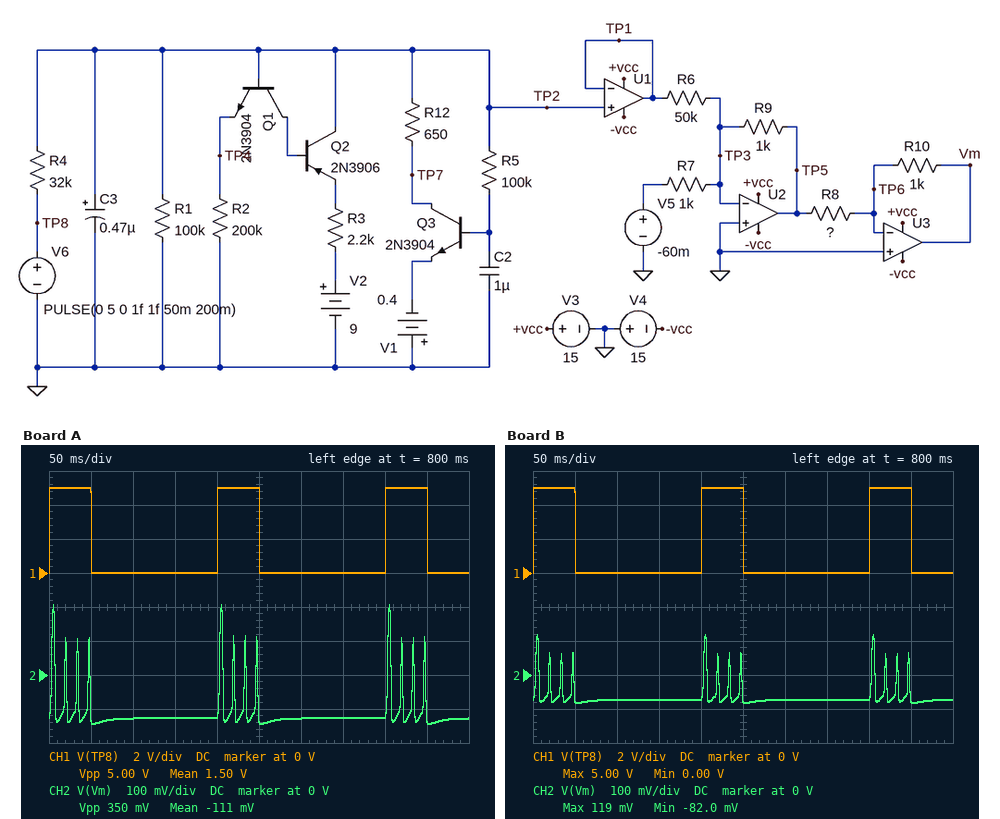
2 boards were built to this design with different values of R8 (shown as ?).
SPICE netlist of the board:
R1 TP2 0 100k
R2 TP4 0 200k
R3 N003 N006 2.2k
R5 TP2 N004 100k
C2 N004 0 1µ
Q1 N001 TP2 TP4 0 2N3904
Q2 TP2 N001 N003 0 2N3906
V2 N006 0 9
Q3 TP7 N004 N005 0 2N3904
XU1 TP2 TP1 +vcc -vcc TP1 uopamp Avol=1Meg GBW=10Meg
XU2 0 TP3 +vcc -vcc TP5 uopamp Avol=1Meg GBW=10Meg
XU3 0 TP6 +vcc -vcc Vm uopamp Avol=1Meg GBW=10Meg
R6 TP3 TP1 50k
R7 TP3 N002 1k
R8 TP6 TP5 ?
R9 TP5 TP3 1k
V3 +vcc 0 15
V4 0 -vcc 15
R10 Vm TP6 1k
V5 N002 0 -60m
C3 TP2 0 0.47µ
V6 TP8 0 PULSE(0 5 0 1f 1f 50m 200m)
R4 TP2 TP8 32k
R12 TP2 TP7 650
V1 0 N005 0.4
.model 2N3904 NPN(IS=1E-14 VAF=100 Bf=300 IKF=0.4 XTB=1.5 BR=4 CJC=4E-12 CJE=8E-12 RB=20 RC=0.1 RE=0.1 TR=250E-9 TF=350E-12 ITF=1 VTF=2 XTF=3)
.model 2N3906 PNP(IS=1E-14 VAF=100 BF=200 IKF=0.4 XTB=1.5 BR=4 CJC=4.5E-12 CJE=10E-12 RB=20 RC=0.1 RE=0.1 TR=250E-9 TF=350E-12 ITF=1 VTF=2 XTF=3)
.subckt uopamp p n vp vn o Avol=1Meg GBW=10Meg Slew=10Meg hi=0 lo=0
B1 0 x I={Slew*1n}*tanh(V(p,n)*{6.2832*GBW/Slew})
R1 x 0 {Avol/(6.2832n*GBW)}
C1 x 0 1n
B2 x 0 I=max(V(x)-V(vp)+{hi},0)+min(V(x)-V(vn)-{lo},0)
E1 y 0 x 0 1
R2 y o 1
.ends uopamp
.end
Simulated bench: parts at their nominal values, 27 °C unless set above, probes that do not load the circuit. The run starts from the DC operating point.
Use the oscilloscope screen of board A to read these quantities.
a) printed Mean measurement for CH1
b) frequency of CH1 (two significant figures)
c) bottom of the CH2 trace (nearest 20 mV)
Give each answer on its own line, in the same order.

1.50 V
5.0 Hz
-140 mV
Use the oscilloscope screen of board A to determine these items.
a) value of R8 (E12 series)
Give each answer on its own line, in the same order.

470 Ω
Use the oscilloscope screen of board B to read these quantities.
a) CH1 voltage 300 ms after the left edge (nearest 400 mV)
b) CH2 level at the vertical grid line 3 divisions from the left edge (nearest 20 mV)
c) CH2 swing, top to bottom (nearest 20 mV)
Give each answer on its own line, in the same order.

0 V
-80 mV
200 mV
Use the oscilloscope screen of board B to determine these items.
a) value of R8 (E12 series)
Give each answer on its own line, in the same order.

820 Ω
